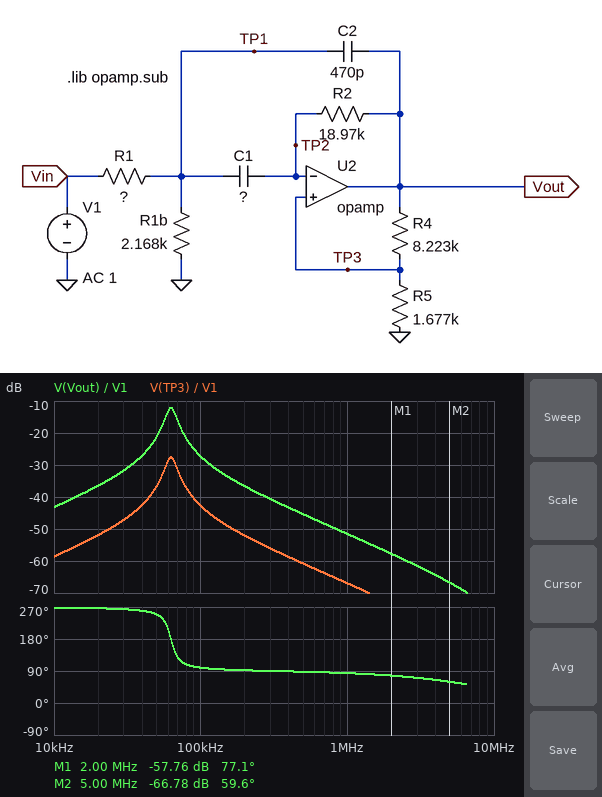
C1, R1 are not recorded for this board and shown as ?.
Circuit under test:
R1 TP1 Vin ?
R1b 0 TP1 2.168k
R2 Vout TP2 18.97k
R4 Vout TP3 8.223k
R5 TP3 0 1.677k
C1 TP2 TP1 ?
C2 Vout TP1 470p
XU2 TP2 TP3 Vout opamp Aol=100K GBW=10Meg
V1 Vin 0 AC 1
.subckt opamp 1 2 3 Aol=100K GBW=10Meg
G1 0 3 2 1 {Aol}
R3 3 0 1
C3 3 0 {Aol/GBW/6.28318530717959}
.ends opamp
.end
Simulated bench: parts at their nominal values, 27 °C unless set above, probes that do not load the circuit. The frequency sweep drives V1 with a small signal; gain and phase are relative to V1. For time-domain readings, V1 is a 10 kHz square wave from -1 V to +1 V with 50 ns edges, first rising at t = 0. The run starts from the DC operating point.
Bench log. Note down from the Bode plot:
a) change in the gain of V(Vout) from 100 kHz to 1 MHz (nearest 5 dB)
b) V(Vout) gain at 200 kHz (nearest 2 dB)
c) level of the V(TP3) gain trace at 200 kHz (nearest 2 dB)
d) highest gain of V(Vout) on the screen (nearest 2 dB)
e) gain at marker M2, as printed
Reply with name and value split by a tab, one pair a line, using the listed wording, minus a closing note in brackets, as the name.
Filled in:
change in the gain of V(Vout) from 100 kHz to 1 MHz	-25 dB
V(Vout) gain at 200 kHz	-36 dB
level of the V(TP3) gain trace at 200 kHz	-52 dB
highest gain of V(Vout) on the screen	-12 dB
gain at marker M2, as printed	-66.78 dB
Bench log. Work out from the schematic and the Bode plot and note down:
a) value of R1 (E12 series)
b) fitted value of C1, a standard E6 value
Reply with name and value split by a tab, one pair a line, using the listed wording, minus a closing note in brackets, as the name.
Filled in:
value of R1	150 kΩ
fitted value of C1, a standard E6 value	330 pF
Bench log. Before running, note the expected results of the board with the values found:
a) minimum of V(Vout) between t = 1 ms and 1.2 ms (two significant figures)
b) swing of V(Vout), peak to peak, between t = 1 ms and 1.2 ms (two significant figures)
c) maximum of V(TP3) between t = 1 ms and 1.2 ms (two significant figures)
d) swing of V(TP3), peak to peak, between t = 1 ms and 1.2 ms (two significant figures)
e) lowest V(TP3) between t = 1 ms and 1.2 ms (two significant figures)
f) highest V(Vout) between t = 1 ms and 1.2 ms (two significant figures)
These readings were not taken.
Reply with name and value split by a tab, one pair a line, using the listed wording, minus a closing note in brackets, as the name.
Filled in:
minimum of V(Vout) between t = 1 ms and 1.2 ms	-65 mV
swing of V(Vout), peak to peak, between t = 1 ms and 1.2 ms	130 mV
maximum of V(TP3) between t = 1 ms and 1.2 ms	11 mV
swing of V(TP3), peak to peak, between t = 1 ms and 1.2 ms	22 mV
lowest V(TP3) between t = 1 ms and 1.2 ms	-11 mV
highest V(Vout) between t = 1 ms and 1.2 ms	65 mV
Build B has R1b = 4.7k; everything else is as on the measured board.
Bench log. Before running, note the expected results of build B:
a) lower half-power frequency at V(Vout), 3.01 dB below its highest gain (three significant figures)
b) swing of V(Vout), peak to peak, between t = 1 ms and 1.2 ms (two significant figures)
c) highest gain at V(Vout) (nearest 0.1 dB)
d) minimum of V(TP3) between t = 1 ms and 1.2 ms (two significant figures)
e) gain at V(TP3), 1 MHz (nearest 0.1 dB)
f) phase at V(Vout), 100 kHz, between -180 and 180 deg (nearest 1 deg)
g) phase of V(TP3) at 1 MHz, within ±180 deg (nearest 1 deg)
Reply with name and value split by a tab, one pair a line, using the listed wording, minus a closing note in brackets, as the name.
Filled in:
lower half-power frequency at V(Vout), 3.01 dB below its highest gain	31.5 kHz
swing of V(Vout), peak to peak, between t = 1 ms and 1.2 ms	160 mV
highest gain at V(Vout)	-20.3 dB
minimum of V(TP3) between t = 1 ms and 1.2 ms	-14 mV
gain at V(TP3), 1 MHz	-66.9 dB
phase at V(Vout), 100 kHz, between -180 and 180 deg	108 deg
phase of V(TP3) at 1 MHz, within ±180 deg	85 deg
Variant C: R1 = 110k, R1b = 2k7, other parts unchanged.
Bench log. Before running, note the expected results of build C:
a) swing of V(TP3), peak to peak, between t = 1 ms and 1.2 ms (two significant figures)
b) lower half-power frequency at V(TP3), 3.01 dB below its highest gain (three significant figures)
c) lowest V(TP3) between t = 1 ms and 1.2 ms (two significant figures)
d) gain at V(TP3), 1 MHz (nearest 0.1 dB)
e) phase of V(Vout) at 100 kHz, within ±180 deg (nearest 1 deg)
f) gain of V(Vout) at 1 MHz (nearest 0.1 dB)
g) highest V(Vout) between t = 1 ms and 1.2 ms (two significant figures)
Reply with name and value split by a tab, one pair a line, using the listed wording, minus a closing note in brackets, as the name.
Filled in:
swing of V(TP3), peak to peak, between t = 1 ms and 1.2 ms	35 mV
lower half-power frequency at V(TP3), 3.01 dB below its highest gain	48.9 kHz
lowest V(TP3) between t = 1 ms and 1.2 ms	-17 mV
gain at V(TP3), 1 MHz	-64.2 dB
phase of V(Vout) at 100 kHz, within ±180 deg	103 deg
gain of V(Vout) at 1 MHz	-48.8 dB
highest V(Vout) between t = 1 ms and 1.2 ms	100 mV
